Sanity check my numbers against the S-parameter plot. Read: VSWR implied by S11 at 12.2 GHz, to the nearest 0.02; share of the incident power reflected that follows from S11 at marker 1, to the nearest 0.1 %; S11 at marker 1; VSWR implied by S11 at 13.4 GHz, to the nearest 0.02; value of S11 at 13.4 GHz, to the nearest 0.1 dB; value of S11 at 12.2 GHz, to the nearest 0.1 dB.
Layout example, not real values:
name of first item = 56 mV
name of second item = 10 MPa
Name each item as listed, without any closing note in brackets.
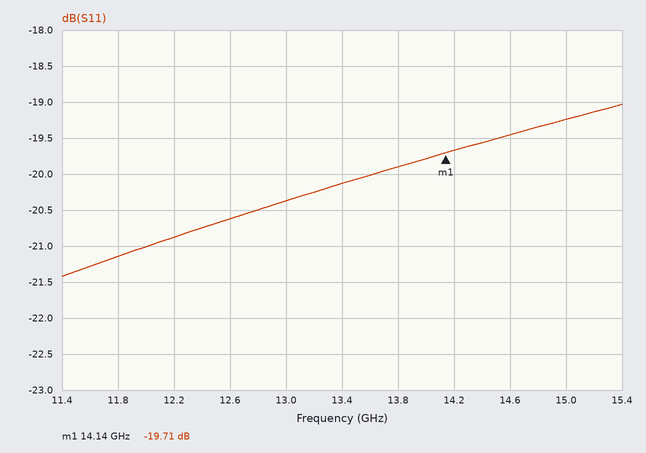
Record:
VSWR implied by S11 at 12.2 GHz, to the nearest 0.02 = 1.20
share of the incident power reflected that follows from S11 at marker 1, to the nearest 0.1 % = 1.1 %
S11 at marker 1 = -19.71 dB
VSWR implied by S11 at 13.4 GHz, to the nearest 0.02 = 1.22
value of S11 at 13.4 GHz, to the nearest 0.1 dB = -20.1 dB
value of S11 at 12.2 GHz, to the nearest 0.1 dB = -20.9 dB
